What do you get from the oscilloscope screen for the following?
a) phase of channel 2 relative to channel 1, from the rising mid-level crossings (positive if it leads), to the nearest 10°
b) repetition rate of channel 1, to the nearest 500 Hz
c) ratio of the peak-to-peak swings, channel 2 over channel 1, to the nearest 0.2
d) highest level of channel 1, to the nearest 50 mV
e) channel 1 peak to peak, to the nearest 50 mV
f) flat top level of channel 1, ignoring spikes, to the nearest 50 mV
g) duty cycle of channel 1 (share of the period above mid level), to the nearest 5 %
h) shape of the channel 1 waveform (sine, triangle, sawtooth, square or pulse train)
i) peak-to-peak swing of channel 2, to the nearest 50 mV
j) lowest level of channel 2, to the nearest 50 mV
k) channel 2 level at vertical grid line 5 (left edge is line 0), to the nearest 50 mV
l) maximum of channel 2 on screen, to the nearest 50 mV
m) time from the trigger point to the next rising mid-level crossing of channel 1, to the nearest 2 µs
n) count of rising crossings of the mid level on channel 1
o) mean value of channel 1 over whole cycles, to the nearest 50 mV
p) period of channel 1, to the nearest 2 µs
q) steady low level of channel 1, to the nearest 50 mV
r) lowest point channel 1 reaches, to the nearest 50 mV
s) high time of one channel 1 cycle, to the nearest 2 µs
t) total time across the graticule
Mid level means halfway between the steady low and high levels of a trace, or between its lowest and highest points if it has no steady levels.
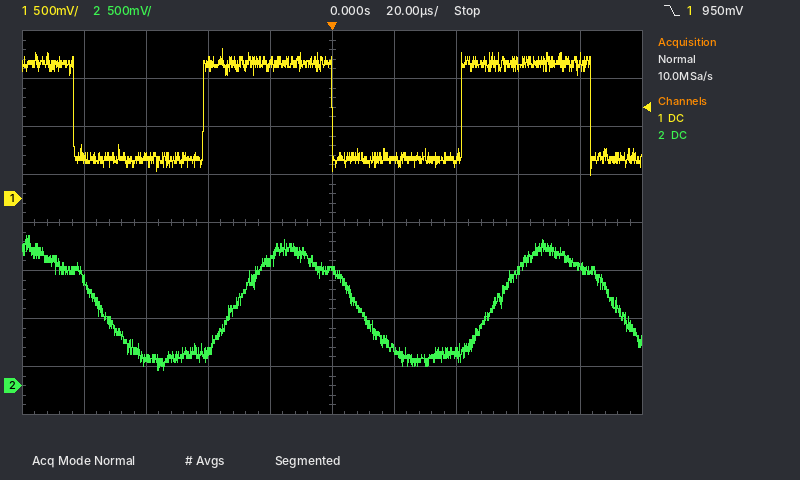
-50°
12.0 kHz
1.0
1.55 V
1.30 V
1.40 V
50 %
square
1.40 V
150 mV
1.20 V
1.55 V
42 µs
2
900 mV
84 µs
400 mV
250 mV
42 µs
200 µs
